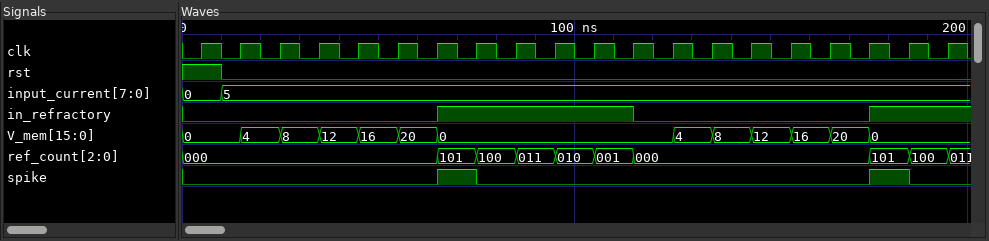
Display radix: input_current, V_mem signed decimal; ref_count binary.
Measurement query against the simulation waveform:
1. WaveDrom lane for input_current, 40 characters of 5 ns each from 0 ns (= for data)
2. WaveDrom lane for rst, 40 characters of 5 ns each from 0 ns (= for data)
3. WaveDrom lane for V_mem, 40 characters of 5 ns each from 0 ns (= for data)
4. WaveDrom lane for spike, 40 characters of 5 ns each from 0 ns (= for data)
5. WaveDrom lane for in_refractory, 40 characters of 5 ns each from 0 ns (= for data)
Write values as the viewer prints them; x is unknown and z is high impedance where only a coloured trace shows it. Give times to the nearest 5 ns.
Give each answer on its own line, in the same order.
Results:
{name: 'input_current', wave: '=.=.....................................', data: '0 5'}
{name: 'rst', wave: '1.0.....................................'}
{name: 'V_mem', wave: '=..=.=.=.=.=.=...........=.=.=.=.=.=....', data: '0 4 8 12 16 20 0 4 8 12 16 20 0'}
{name: 'spike', wave: '0............1.0...................1.0..'}
{name: 'in_refractory', wave: '0............1.........0...........1....'}
